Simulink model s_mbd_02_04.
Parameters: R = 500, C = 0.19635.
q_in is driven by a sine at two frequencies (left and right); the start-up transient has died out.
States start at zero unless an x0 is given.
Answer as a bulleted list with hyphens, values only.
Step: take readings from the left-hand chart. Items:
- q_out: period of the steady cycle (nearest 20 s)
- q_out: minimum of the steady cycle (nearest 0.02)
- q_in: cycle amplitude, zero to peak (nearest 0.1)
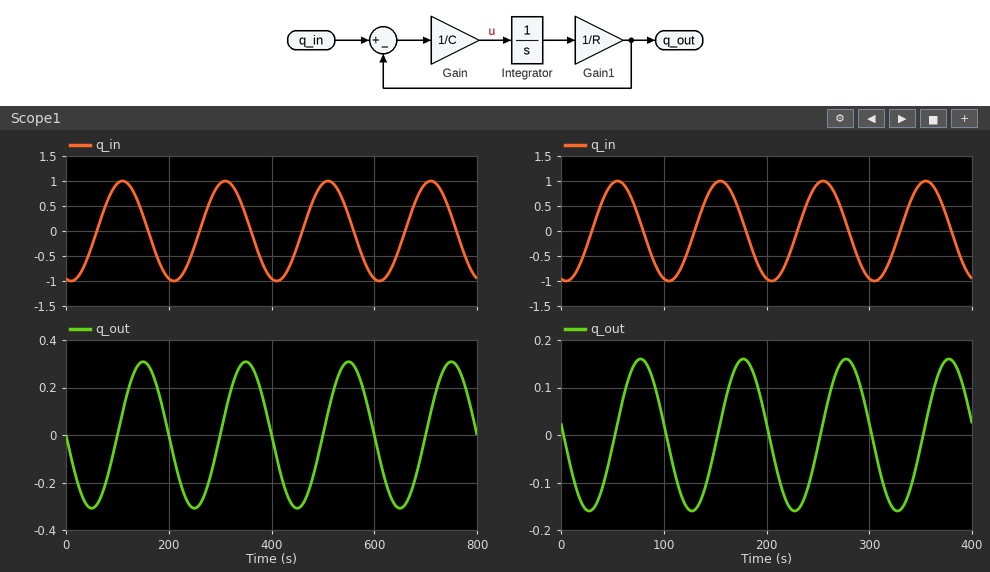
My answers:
- 200 s
- -0.30
- 1.0
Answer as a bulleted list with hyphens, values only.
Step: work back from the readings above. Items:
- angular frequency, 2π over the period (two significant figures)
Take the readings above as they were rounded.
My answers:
- 0.031 rad/s
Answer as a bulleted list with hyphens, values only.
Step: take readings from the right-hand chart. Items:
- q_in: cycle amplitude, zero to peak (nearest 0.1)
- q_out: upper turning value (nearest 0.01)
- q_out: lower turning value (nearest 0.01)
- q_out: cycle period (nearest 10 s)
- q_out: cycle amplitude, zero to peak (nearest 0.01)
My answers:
- 1.0
- 0.16
- -0.16
- 100 s
- 0.16
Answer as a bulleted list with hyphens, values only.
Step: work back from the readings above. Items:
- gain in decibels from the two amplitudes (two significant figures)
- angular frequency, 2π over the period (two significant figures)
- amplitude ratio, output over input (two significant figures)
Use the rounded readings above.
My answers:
- -16 dB
- 0.063 rad/s
- 0.16
